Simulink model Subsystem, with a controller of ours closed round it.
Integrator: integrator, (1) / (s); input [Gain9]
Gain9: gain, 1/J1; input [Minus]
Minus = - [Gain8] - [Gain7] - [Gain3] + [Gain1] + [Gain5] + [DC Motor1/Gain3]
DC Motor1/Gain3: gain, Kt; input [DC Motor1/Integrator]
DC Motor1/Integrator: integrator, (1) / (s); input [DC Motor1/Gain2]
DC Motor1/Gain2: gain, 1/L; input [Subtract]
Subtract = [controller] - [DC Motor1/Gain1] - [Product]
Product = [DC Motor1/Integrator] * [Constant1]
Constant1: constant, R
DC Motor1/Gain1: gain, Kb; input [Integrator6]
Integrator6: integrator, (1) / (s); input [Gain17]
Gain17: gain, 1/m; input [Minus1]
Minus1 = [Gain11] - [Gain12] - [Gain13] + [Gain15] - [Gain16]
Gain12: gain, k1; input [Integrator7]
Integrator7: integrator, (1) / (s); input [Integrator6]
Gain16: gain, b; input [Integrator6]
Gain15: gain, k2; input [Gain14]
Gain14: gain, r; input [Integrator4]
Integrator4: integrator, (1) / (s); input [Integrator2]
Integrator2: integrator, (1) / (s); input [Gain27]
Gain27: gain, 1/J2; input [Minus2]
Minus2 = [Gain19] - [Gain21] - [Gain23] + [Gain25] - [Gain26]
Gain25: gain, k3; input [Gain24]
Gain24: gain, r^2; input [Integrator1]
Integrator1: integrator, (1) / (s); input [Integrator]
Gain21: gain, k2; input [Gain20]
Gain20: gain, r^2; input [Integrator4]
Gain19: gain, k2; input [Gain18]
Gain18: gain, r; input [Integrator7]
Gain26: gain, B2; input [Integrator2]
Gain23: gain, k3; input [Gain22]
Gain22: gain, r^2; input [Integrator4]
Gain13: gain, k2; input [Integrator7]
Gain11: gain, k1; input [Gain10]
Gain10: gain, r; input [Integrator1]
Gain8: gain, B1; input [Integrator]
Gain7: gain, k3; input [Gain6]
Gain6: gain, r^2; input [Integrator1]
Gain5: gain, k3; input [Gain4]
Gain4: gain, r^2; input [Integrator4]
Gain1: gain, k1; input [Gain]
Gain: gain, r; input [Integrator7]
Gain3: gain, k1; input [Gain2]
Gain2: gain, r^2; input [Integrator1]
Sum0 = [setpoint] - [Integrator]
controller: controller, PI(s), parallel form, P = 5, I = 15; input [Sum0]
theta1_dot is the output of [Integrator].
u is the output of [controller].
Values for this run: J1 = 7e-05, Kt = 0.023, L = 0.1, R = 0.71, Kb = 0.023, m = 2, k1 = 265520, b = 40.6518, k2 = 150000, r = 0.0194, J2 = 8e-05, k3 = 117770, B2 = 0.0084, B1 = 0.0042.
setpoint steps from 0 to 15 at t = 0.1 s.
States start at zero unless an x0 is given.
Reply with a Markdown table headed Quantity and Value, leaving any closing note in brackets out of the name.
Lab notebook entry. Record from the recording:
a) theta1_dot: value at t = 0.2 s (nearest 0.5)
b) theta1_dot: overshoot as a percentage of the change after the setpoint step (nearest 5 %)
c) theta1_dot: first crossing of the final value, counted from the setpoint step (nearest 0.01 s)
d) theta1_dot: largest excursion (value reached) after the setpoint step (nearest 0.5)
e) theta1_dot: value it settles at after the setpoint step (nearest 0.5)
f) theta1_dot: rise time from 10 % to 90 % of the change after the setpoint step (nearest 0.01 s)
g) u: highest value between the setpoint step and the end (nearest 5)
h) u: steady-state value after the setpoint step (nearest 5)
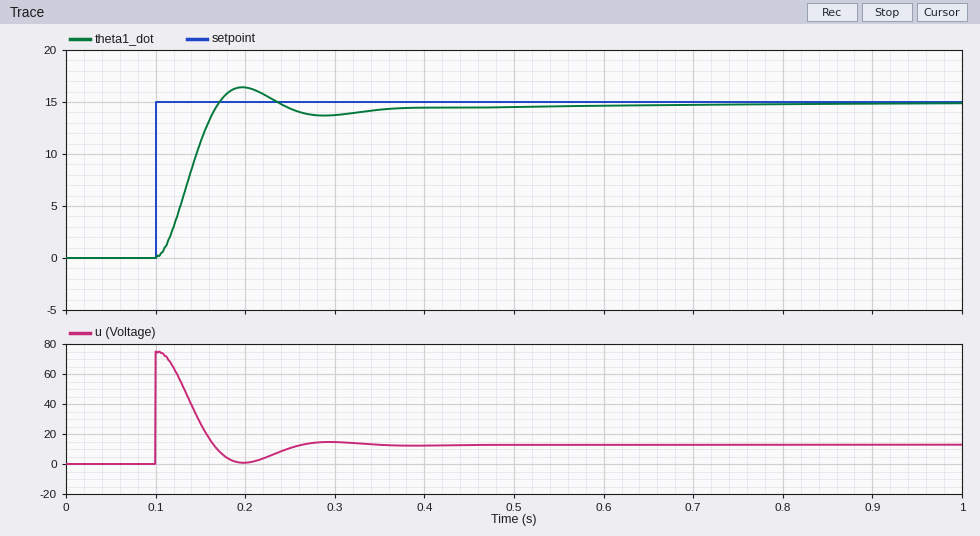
| Quantity | Value |
|---|---|
| theta1_dot: value at t = 0.2 s | 16.5 |
| theta1_dot: overshoot as a percentage of the change after the setpoint step | 10 % |
| theta1_dot: first crossing of the final value, counted from the setpoint step | 0.07 s |
| theta1_dot: largest excursion (value reached) after the setpoint step | 16.5 |
| theta1_dot: value it settles at after the setpoint step | 15.0 |
| theta1_dot: rise time from 10 % to 90 % of the change after the setpoint step | 0.05 s |
| u: highest value between the setpoint step and the end | 75 |
| u: steady-state value after the setpoint step | 15 |
